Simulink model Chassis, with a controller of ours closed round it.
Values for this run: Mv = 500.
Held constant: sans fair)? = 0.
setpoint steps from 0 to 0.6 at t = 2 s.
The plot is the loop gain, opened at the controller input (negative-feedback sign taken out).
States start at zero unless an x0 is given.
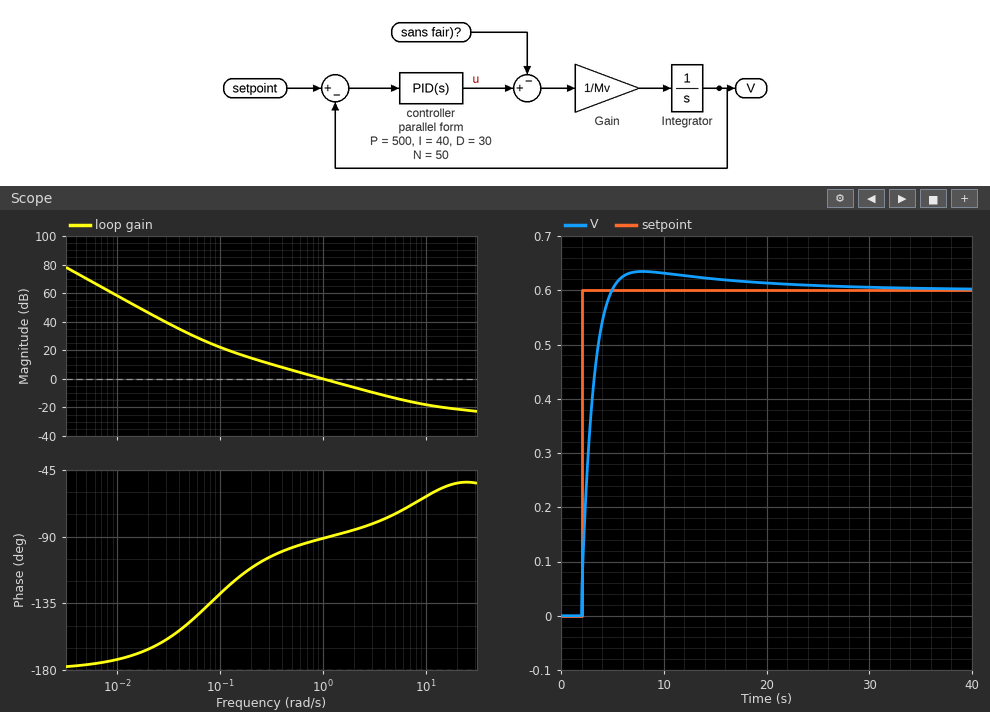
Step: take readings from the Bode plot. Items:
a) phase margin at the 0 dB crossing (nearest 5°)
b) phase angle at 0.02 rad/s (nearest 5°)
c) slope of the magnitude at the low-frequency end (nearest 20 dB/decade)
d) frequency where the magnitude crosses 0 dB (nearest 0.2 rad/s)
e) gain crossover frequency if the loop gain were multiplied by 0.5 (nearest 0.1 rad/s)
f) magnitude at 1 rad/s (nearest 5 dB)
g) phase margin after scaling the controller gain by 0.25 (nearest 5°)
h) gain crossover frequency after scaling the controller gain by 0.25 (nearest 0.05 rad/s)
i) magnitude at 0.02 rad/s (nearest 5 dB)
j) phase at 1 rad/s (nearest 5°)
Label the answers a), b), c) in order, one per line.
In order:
a) 90°
b) -165°
c) -40 dB/decade
d) 1.0 rad/s
e) 0.5 rad/s
f) 0 dB
g) 75°
h) 0.25 rad/s
i) 45 dB
j) -90°
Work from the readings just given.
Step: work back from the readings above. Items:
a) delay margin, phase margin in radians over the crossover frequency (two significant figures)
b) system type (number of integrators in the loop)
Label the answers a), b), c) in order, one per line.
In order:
a) 1.6 s
b) 2
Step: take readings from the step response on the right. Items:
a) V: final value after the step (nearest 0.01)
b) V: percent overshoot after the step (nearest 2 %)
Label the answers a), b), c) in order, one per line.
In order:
a) 0.60
b) 6 %
